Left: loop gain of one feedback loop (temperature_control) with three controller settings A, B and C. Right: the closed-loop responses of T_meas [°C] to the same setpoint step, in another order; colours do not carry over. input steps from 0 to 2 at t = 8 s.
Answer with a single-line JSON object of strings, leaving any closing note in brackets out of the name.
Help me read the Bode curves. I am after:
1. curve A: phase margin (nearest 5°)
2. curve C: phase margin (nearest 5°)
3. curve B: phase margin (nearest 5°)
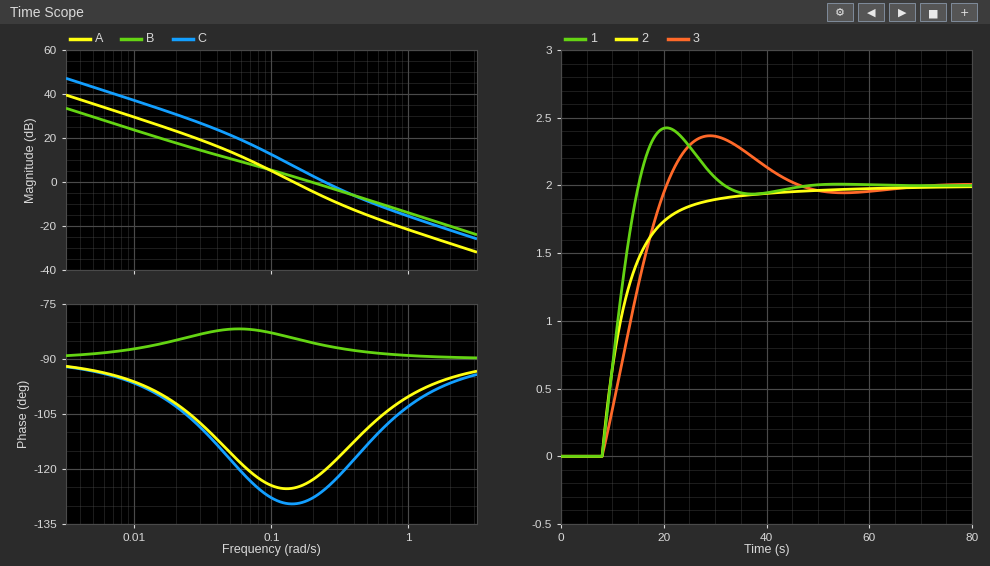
{"curve A: phase margin": "55°", "curve C: phase margin": "55°", "curve B: phase margin": "95°"}
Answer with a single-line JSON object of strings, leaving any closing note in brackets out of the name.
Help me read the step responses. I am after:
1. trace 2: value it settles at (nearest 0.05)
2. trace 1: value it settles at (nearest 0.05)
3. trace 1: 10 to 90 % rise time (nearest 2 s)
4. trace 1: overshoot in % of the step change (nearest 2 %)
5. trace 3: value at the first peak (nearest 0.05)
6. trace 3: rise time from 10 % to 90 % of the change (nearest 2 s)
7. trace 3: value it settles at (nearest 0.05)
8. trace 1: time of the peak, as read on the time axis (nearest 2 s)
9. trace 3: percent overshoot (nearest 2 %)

{"trace 2: value it settles at": "2.00", "trace 1: value it settles at": "2.00", "trace 1: 10 to 90 % rise time": "6 s", "trace 1: overshoot in % of the step change": "22 %", "trace 3: value at the first peak": "2.35", "trace 3: rise time from 10 % to 90 % of the change": "10 s", "trace 3: value it settles at": "2.00", "trace 1: time of the peak, as read on the time axis": "20 s", "trace 3: percent overshoot": "18 %"}
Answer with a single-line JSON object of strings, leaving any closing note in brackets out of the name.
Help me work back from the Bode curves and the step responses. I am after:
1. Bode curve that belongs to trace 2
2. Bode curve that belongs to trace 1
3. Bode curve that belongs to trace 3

{"Bode curve that belongs to trace 2": "B", "Bode curve that belongs to trace 1": "C", "Bode curve that belongs to trace 3": "A"}
